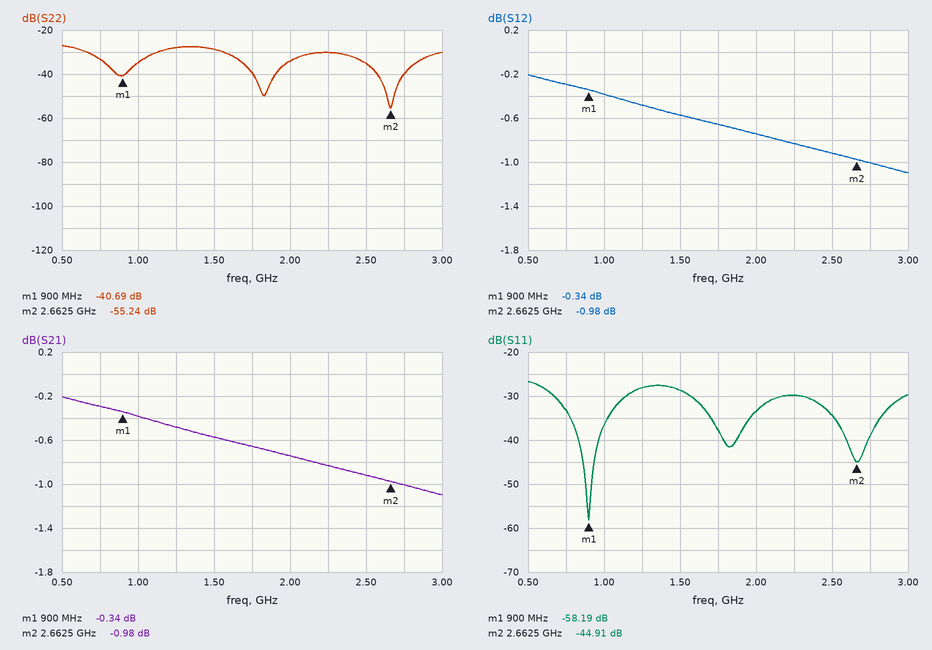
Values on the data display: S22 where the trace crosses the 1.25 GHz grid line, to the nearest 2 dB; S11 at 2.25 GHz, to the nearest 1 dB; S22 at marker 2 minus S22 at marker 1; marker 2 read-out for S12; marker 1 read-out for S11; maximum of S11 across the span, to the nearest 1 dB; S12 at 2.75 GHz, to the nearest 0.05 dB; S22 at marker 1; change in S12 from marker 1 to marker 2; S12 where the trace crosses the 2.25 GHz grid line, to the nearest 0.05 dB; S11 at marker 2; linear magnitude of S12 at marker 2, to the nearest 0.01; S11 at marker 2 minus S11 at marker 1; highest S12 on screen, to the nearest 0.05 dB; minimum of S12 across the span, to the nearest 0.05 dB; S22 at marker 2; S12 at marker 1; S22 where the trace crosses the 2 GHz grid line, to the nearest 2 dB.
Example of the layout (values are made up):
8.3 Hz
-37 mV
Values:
-28 dB
-30 dB
-14.55 dB
-0.98 dB
-58.19 dB
-27 dB
-1.00 dB
-40.69 dB
-0.64 dB
-0.85 dB
-44.91 dB
0.89
13.28 dB
-0.20 dB
-1.10 dB
-55.24 dB
-0.34 dB
-34 dB
